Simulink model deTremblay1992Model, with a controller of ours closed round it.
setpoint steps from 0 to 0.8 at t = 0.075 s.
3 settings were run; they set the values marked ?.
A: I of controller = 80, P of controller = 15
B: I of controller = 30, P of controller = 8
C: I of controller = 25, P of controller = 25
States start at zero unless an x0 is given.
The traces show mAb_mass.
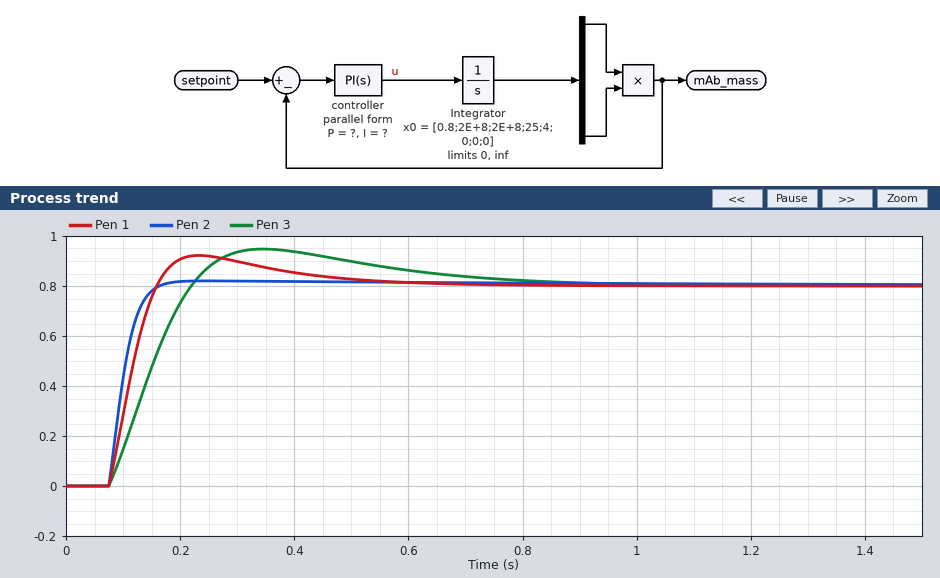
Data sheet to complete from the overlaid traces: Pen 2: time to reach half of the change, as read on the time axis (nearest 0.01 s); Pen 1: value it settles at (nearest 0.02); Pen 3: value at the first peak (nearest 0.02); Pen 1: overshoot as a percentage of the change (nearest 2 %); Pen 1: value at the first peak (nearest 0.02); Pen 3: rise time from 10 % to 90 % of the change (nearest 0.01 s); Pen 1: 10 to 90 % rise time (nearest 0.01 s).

0.10 s
0.80
0.94
16 %
0.92
0.11 s
0.06 s
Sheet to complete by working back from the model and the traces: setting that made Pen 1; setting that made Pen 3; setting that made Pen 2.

A
B
C
